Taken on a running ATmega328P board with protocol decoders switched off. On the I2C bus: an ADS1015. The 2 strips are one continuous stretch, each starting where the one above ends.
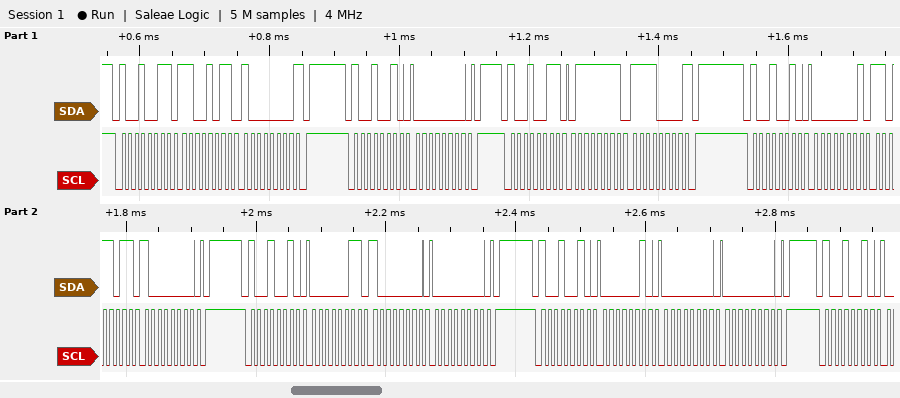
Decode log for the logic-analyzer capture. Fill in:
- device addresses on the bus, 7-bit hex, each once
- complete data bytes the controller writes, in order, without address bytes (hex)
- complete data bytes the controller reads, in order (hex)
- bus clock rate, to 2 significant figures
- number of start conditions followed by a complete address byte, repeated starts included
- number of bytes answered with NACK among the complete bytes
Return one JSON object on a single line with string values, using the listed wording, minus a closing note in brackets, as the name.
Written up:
{"device addresses on the bus, 7-bit hex, each once": "0x49", "complete data bytes the controller writes, in order, without address bytes": "00 01 DB 80 03 80 00 02 00 00", "complete data bytes the controller reads, in order": "CB 80 7F F0", "bus clock rate, to 2 significant figures": "100 kHz", "number of start conditions followed by a complete address byte, repeated starts included": "7", "number of bytes answered with NACK among the complete bytes": "2"}
